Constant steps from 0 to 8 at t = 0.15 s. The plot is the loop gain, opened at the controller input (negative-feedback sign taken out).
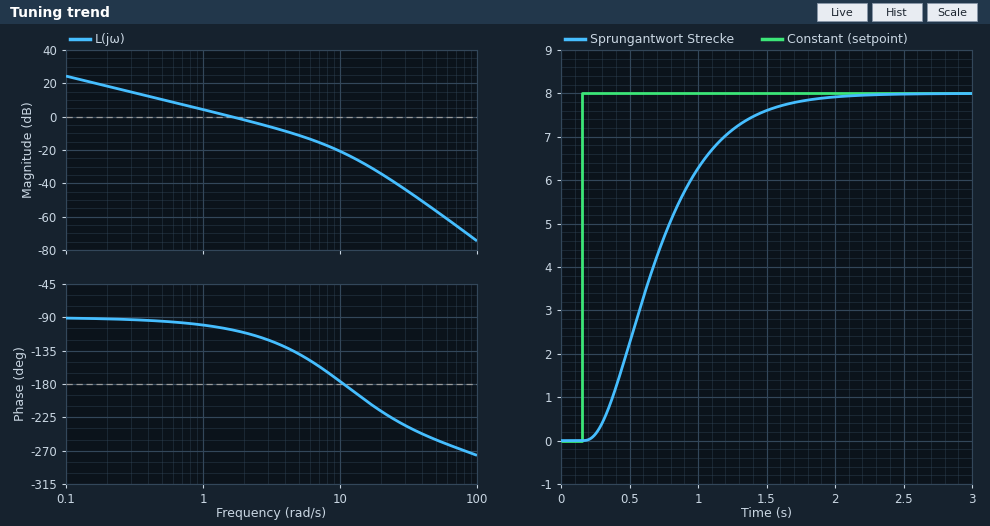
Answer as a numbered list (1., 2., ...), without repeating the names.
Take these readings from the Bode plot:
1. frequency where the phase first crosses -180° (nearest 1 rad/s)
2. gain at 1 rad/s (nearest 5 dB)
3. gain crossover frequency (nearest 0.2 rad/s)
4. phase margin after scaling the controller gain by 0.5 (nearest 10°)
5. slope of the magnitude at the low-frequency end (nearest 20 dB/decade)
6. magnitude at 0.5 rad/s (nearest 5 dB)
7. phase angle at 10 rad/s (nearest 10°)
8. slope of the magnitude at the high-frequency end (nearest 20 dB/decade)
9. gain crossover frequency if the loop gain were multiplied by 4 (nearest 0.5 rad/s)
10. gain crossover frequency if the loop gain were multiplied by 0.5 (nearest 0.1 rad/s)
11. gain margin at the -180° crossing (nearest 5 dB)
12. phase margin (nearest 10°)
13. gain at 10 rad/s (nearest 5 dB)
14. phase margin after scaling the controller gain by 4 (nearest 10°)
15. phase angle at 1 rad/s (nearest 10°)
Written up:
1. 11 rad/s
2. 5 dB
3. 1.6 rad/s
4. 80°
5. -20 dB/decade
6. 10 dB
7. -180°
8. -60 dB/decade
9. 5.5 rad/s
10. 0.8 rad/s
11. 20 dB
12. 70°
13. -20 dB
14. 40°
15. -100°
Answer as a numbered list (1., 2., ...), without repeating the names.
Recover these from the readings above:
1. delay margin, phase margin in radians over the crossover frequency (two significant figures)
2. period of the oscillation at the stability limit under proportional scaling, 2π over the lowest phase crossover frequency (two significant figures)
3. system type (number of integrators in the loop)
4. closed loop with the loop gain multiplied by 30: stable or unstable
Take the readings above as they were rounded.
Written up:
1. 0.76 s
2. 0.57 s
3. 1
4. unstable
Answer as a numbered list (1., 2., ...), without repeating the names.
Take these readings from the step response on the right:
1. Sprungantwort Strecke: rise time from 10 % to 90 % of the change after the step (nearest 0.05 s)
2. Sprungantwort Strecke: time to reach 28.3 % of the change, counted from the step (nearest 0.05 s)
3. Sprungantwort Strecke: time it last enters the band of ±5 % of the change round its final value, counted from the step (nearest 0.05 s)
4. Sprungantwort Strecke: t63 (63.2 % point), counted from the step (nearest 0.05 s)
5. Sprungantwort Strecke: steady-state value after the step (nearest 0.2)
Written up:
1. 0.90 s
2. 0.35 s
3. 1.35 s
4. 0.65 s
5. 8.0
